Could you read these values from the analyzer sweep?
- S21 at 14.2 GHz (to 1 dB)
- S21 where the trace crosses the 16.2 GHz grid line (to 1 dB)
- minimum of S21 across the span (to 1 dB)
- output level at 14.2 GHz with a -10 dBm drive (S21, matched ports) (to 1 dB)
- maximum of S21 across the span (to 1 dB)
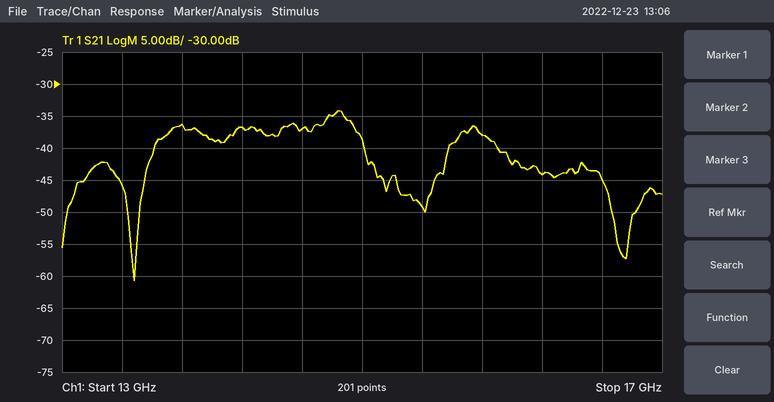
-37 dB
-44 dB
-61 dB
-47 dBm
-34 dB
